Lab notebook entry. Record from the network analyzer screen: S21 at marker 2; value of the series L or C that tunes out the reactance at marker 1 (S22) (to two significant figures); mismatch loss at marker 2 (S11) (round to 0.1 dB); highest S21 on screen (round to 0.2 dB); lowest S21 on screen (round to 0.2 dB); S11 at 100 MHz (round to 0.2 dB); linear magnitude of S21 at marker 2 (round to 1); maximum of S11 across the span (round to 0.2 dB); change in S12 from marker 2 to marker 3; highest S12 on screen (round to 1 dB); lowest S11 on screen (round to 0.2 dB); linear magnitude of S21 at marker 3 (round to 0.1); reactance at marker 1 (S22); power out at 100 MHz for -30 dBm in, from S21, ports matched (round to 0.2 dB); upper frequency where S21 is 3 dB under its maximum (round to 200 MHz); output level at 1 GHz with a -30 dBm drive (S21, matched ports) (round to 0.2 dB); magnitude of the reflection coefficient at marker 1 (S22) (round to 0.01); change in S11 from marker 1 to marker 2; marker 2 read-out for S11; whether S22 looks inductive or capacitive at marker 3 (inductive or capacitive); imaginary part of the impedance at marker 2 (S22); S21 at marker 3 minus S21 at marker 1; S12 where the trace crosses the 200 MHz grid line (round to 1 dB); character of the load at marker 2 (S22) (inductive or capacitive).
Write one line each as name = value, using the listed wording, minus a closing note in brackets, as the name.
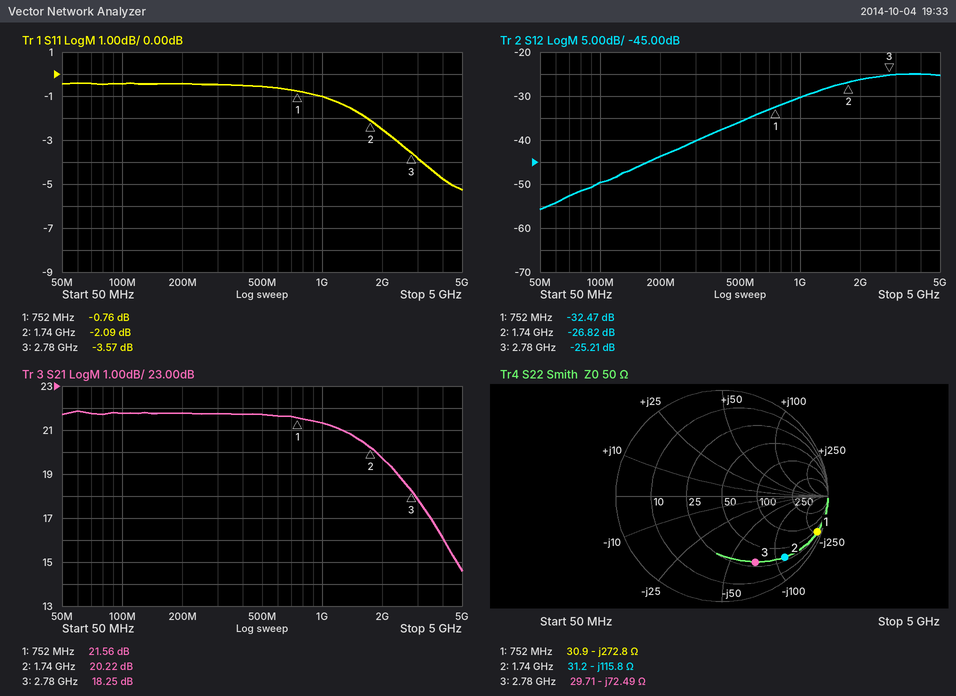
S21 at marker 2 = 20.22 dB
value of the series L or C that tunes out the reactance at marker 1 (S22) = 58 nH
mismatch loss at marker 2 (S11) = 4.2 dB
highest S21 on screen = 21.8 dB
lowest S21 on screen = 14.6 dB
S11 at 100 MHz = -0.4 dB
linear magnitude of S21 at marker 2 = 10
maximum of S11 across the span = -0.4 dB
change in S12 from marker 2 to marker 3 = 1.61 dB
highest S12 on screen = -25 dB
lowest S11 on screen = -5.2 dB
linear magnitude of S21 at marker 3 = 8.2
reactance at marker 1 = -272.8 Ω
power out at 100 MHz for -30 dBm in, from S21, ports matched = -8.2 dBm
upper frequency where S21 is 3 dB under its maximum = 2.4 GHz
output level at 1 GHz with a -30 dBm drive (S21, matched ports) = -8.6 dBm
magnitude of the reflection coefficient at marker 1 (S22) = 0.96
change in S11 from marker 1 to marker 2 = -1.33 dB
marker 2 read-out for S11 = -2.09 dB
whether S22 looks inductive or capacitive at marker 3 = capacitive
imaginary part of the impedance at marker 2 = -115.8 Ω
S21 at marker 3 minus S21 at marker 1 = -3.31 dB
S12 where the trace crosses the 200 MHz grid line = -44 dB
character of the load at marker 2 (S22) = capacitive
